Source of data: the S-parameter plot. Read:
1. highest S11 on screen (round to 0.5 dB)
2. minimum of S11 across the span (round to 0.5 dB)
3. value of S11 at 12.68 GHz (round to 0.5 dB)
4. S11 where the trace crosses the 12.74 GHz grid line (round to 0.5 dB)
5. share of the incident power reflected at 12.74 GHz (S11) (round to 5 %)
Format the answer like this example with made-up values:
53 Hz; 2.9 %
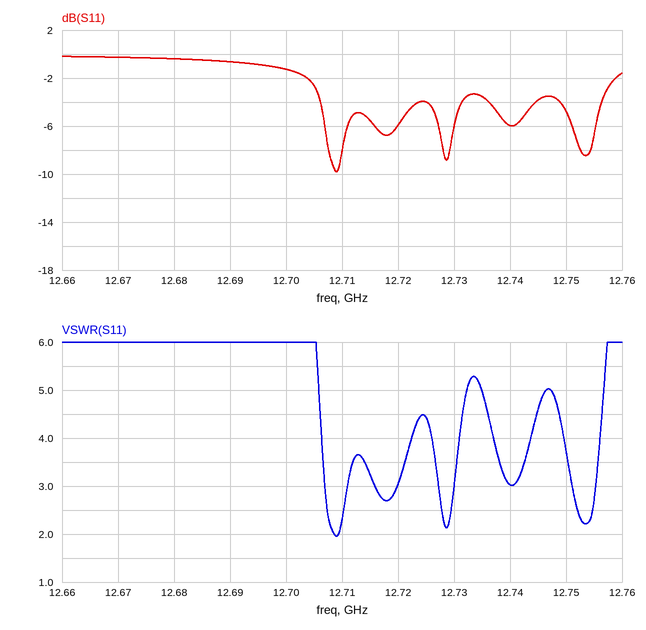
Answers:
0.0 dB; -10.0 dB; -0.5 dB; -6.0 dB; 25 %
